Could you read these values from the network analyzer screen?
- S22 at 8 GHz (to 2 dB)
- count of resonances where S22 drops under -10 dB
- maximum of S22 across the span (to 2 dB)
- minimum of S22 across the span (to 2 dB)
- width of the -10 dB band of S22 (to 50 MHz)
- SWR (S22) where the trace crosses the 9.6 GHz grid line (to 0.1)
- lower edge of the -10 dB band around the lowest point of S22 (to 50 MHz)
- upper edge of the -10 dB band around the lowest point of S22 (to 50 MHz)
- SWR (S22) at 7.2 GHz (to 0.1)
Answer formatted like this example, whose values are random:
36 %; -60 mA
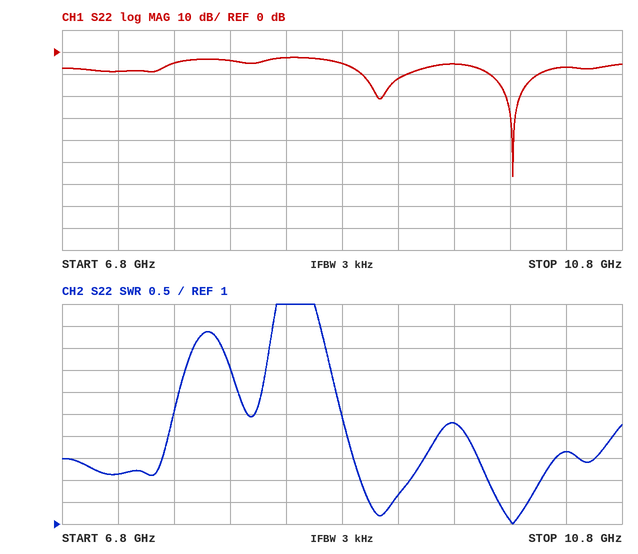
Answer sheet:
-4 dB; 2; -2 dB; -56 dB; 350 MHz; 3.3; 9.85 GHz; 10.20 GHz; 2.1
